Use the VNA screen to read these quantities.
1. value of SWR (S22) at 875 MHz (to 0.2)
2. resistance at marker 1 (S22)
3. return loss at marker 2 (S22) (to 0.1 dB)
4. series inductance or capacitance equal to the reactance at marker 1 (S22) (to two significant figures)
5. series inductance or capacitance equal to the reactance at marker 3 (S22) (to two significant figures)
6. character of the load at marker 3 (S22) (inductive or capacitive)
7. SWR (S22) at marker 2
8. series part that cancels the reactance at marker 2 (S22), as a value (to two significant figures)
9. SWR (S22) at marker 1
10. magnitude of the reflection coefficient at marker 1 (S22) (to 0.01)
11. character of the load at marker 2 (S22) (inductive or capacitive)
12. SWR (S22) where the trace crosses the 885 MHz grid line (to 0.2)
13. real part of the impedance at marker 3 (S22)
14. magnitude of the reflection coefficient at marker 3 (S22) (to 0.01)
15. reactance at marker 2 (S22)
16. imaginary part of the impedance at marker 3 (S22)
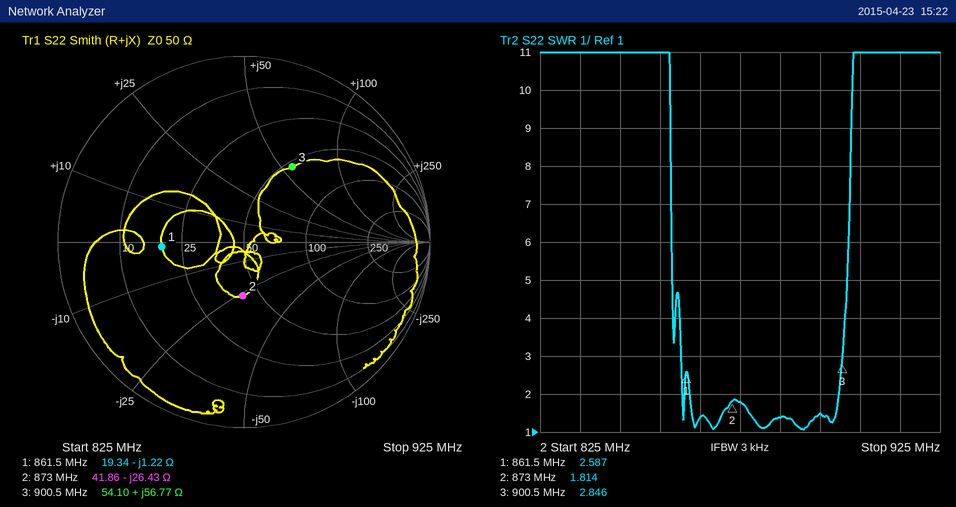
1.8
19.34 Ω
10.8 dB
150 pF
10 nH
inductive
1.814
4.8 nH
2.587
0.44
capacitive
1.4
54.10 Ω
0.48
-26.43 Ω
+56.77 Ω
